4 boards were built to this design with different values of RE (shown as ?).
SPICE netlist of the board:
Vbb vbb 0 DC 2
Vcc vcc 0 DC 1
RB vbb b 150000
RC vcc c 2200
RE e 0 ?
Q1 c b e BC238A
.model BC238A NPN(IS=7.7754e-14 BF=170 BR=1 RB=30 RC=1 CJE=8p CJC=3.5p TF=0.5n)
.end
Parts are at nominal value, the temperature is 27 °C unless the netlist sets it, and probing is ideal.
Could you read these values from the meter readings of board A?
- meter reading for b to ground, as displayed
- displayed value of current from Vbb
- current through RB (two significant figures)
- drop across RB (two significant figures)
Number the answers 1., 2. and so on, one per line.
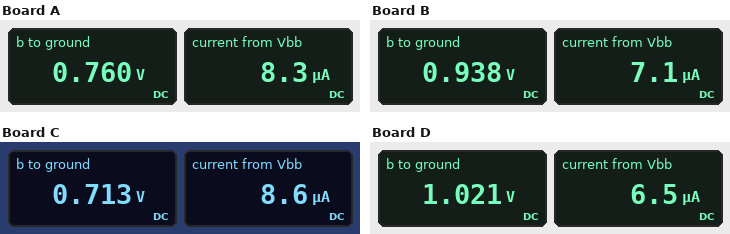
1. 0.760 V
2. 8.3 µA
3. 8.3 µA
4. 1.2 V
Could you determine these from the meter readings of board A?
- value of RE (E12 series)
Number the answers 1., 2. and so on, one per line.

1. 560 Ω
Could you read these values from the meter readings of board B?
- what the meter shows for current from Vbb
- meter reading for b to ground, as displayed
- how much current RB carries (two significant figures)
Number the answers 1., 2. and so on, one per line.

1. 7.1 µA
2. 0.938 V
3. 7.1 µA
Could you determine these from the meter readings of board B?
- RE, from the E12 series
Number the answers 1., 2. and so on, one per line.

1. 1.5 kΩ
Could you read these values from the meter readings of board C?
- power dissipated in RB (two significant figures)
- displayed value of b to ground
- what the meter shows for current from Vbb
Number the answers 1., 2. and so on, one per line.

1. 11 µW
2. 0.713 V
3. 8.6 µA
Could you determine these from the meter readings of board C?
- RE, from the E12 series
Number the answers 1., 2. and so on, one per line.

1. 390 Ω
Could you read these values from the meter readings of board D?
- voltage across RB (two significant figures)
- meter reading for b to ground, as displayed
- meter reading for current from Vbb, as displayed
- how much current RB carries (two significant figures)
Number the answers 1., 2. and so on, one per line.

1. 980 mV
2. 1.021 V
3. 6.5 µA
4. 6.5 µA
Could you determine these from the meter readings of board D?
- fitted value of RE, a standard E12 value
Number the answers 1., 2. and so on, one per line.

1. 2.2 kΩ
